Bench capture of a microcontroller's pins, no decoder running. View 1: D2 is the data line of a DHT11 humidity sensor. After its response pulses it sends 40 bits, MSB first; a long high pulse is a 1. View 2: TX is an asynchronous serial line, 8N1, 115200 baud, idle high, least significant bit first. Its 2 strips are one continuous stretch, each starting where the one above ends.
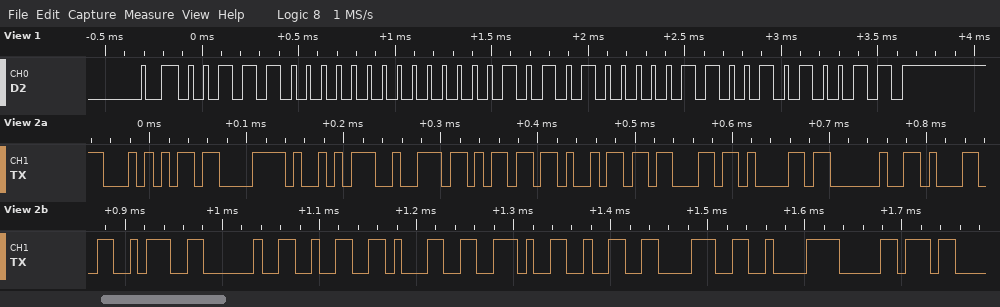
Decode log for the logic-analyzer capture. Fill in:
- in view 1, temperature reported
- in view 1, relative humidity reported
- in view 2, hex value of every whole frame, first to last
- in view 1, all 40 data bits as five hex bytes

21.6 °C
56 %
0x54 0xC3 0xA9 0x72 0x6D 0x69 0x63 0x61 0x20 0x31 0x3A 0x20 0x32 0x31 0x2E 0x32 0x38 0xC2 0xB0
38 00 15 06 53
